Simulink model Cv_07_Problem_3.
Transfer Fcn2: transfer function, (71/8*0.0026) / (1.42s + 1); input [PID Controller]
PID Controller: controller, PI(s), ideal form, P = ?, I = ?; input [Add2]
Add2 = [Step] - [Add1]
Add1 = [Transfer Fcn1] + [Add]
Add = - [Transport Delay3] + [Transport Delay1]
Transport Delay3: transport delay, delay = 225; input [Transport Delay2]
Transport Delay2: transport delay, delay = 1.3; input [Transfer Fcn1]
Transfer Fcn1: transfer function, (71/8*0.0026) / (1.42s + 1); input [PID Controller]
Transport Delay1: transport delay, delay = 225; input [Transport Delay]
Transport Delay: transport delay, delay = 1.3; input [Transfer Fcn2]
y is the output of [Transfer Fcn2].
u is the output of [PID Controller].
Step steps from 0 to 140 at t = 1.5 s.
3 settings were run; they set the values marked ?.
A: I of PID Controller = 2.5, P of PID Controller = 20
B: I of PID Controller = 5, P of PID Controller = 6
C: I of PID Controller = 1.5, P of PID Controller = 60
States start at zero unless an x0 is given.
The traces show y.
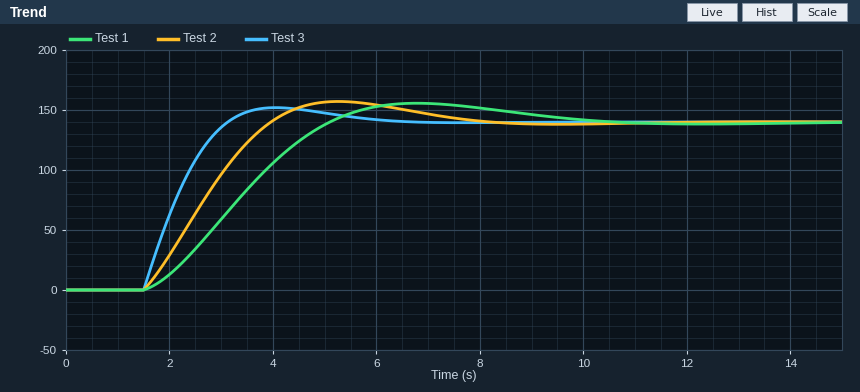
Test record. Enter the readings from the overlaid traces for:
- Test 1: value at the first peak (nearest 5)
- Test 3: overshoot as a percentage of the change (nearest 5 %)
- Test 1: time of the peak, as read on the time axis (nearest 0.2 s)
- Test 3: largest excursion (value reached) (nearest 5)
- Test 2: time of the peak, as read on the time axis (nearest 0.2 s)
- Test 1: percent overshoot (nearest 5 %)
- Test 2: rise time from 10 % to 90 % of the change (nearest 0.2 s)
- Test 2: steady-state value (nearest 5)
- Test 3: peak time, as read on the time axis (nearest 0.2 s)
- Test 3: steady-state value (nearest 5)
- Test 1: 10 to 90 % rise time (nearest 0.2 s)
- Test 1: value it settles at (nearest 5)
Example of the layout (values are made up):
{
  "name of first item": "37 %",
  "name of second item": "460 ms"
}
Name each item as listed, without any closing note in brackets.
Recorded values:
{
  "Test 1: value at the first peak": "155",
  "Test 3: overshoot as a percentage of the change": "10 %",
  "Test 1: time of the peak, as read on the time axis": "6.8 s",
  "Test 3: largest excursion (value reached)": "150",
  "Test 2: time of the peak, as read on the time axis": "5.2 s",
  "Test 1: percent overshoot": "10 %",
  "Test 2: rise time from 10 % to 90 % of the change": "1.8 s",
  "Test 2: steady-state value": "140",
  "Test 3: peak time, as read on the time axis": "4.0 s",
  "Test 3: steady-state value": "140",
  "Test 1: 10 to 90 % rise time": "2.6 s",
  "Test 1: value it settles at": "140"
}
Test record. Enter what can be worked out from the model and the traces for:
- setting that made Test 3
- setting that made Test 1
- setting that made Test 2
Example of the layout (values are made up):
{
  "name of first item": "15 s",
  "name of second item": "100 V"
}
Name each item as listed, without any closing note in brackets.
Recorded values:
{
  "setting that made Test 3": "C",
  "setting that made Test 1": "B",
  "setting that made Test 2": "A"
}
